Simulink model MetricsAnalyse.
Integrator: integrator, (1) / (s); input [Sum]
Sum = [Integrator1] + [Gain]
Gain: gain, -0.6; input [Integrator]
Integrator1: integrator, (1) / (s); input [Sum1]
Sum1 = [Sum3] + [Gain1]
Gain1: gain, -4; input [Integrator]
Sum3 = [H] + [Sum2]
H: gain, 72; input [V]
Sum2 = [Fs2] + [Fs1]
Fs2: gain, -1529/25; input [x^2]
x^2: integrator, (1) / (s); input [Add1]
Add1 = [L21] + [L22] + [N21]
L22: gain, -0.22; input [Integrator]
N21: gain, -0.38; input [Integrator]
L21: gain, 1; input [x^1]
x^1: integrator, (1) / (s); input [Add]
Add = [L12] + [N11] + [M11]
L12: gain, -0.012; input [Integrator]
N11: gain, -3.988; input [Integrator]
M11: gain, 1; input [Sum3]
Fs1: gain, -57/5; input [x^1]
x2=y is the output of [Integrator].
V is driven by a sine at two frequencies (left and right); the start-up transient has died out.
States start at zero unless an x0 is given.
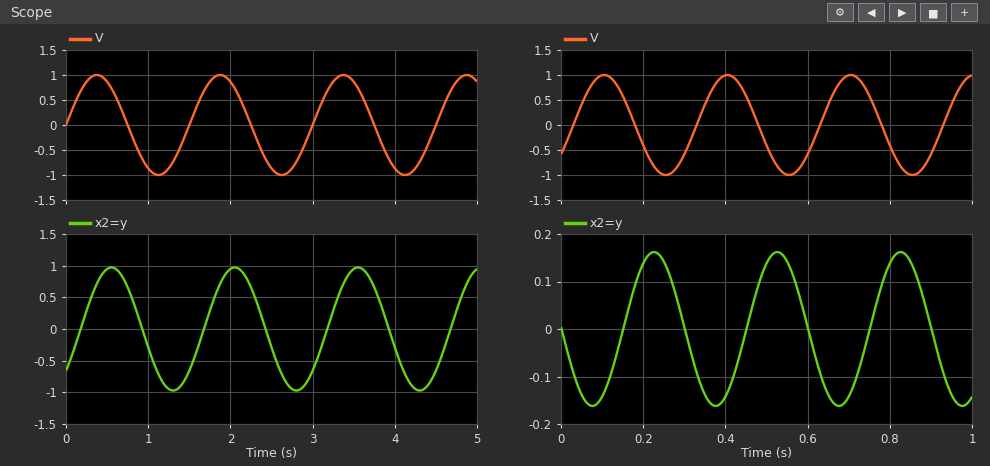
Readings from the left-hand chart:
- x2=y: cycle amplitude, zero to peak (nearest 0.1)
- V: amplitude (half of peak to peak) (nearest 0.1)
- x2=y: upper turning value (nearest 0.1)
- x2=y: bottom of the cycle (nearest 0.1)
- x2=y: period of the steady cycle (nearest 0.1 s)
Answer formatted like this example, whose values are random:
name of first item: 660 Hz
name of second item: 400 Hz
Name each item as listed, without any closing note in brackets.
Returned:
x2=y: cycle amplitude, zero to peak: 1.0
V: amplitude (half of peak to peak): 1.0
x2=y: upper turning value: 1.0
x2=y: bottom of the cycle: -1.0
x2=y: period of the steady cycle: 1.5 s
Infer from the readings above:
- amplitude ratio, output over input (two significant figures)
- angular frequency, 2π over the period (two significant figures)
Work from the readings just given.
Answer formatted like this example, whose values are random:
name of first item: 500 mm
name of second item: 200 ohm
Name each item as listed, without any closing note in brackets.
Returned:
amplitude ratio, output over input: 1.0
angular frequency, 2π over the period: 4.2 rad/s
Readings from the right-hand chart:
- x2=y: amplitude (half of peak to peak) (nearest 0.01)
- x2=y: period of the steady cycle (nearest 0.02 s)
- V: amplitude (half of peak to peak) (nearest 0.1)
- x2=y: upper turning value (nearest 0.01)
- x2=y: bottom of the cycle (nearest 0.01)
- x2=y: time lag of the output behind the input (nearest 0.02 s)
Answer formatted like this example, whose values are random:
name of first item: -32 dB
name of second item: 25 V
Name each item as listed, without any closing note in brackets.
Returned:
x2=y: amplitude (half of peak to peak): 0.16
x2=y: period of the steady cycle: 0.30 s
V: amplitude (half of peak to peak): 1.0
x2=y: upper turning value: 0.16
x2=y: bottom of the cycle: -0.16
x2=y: time lag of the output behind the input: 0.12 s
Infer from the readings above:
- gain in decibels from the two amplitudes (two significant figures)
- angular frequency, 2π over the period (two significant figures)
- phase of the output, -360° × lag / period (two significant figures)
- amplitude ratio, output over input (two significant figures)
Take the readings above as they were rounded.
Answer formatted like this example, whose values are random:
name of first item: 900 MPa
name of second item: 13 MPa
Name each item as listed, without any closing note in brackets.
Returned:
gain in decibels from the two amplitudes: -16 dB
angular frequency, 2π over the period: 21 rad/s
phase of the output, -360° × lag / period: -140°
amplitude ratio, output over input: 0.16
